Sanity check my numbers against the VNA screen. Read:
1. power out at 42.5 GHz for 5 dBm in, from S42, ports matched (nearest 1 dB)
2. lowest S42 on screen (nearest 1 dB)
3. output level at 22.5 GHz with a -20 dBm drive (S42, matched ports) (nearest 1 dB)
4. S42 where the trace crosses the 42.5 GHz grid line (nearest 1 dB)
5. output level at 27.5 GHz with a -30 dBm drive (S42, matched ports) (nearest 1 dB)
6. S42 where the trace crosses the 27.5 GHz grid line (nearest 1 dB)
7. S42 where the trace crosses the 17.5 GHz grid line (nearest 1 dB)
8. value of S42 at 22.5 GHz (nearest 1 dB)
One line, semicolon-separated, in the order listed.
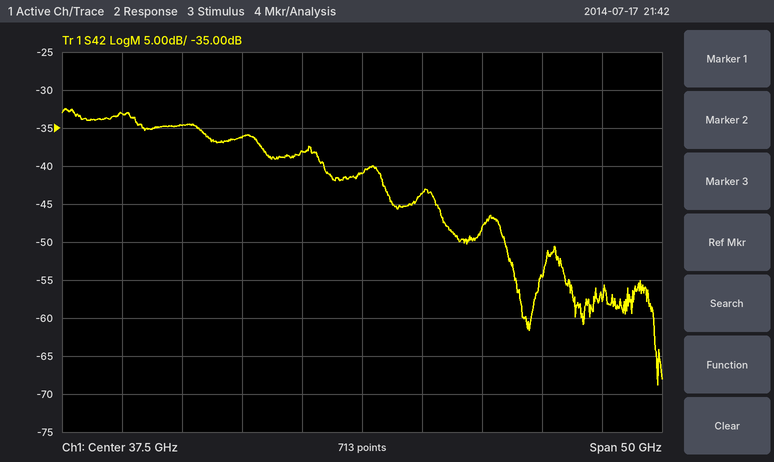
-39 dBm; -69 dB; -55 dBm; -44 dB; -66 dBm; -36 dB; -33 dB; -35 dB
